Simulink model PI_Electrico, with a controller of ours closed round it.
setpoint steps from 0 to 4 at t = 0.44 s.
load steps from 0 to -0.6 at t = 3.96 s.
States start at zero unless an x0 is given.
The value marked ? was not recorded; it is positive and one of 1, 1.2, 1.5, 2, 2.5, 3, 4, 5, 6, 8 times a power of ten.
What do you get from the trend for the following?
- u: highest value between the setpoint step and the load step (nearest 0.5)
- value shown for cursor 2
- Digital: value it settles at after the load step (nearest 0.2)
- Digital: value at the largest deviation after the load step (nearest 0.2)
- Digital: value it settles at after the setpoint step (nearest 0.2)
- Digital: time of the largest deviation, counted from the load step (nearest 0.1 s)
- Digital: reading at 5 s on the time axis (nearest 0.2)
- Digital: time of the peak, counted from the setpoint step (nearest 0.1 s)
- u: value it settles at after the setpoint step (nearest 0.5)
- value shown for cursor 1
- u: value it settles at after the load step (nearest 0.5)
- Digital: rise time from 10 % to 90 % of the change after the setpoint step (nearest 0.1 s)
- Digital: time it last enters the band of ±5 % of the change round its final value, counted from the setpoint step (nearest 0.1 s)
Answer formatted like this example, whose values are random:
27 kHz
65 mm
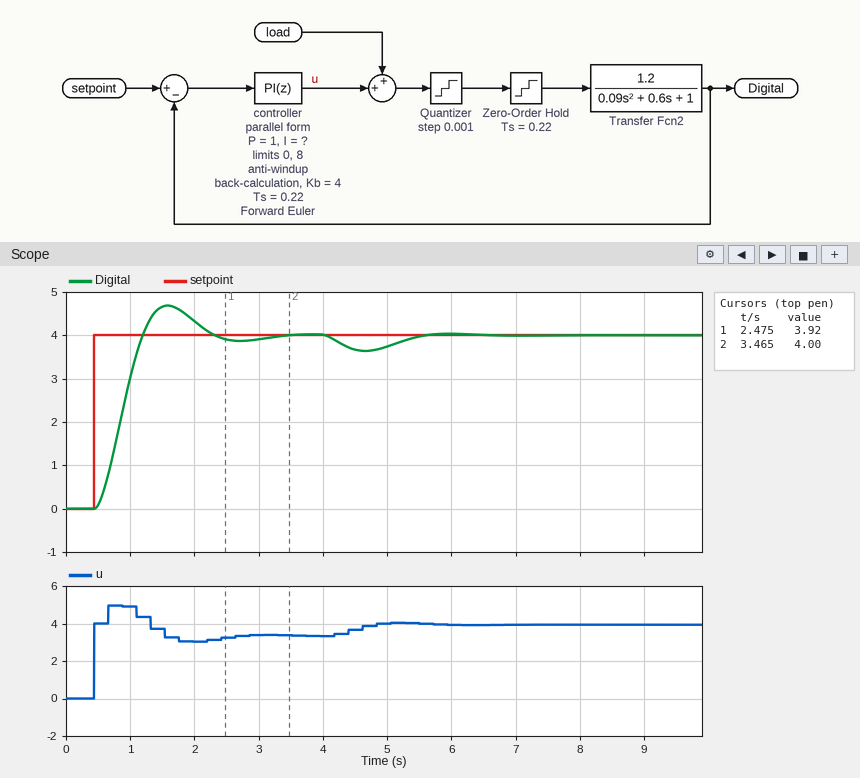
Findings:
5.0
4.00
4.0
3.6
4.0
0.7 s
3.8
1.1 s
3.5
3.92
4.0
0.5 s
1.7 s
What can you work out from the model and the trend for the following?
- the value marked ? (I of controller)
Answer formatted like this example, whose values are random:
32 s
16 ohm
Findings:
2
